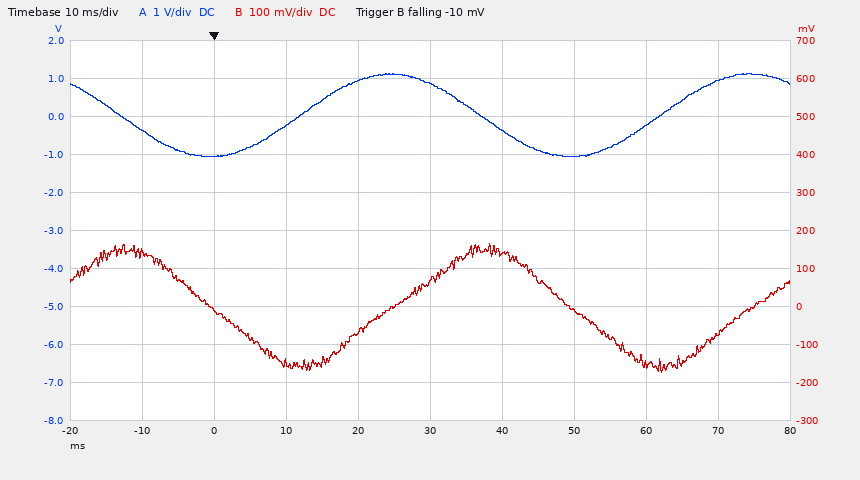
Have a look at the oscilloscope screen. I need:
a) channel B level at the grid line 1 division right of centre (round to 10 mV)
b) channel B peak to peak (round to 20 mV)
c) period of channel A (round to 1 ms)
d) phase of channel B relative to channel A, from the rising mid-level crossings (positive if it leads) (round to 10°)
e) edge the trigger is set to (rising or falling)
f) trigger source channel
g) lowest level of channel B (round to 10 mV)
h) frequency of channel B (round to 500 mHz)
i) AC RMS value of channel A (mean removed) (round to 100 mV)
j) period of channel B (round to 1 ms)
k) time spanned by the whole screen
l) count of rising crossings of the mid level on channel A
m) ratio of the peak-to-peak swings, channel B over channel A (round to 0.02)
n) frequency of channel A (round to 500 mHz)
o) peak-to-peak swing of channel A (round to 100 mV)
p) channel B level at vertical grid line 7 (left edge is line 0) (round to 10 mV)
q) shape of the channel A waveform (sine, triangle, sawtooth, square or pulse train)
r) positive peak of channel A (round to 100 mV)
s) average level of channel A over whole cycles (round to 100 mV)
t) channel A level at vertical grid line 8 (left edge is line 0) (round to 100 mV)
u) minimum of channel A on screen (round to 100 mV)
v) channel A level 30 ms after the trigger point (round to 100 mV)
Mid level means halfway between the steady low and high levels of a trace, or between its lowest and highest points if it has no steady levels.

140 mV
340 mV
50 ms
-90°
falling
channel B
-170 mV
20.0 Hz
800 mV
50 ms
100 ms
2
0.16
20.0 Hz
2.2 V
-10 mV
sine
1.1 V
0.0 V
-200 mV
-1.1 V
900 mV
